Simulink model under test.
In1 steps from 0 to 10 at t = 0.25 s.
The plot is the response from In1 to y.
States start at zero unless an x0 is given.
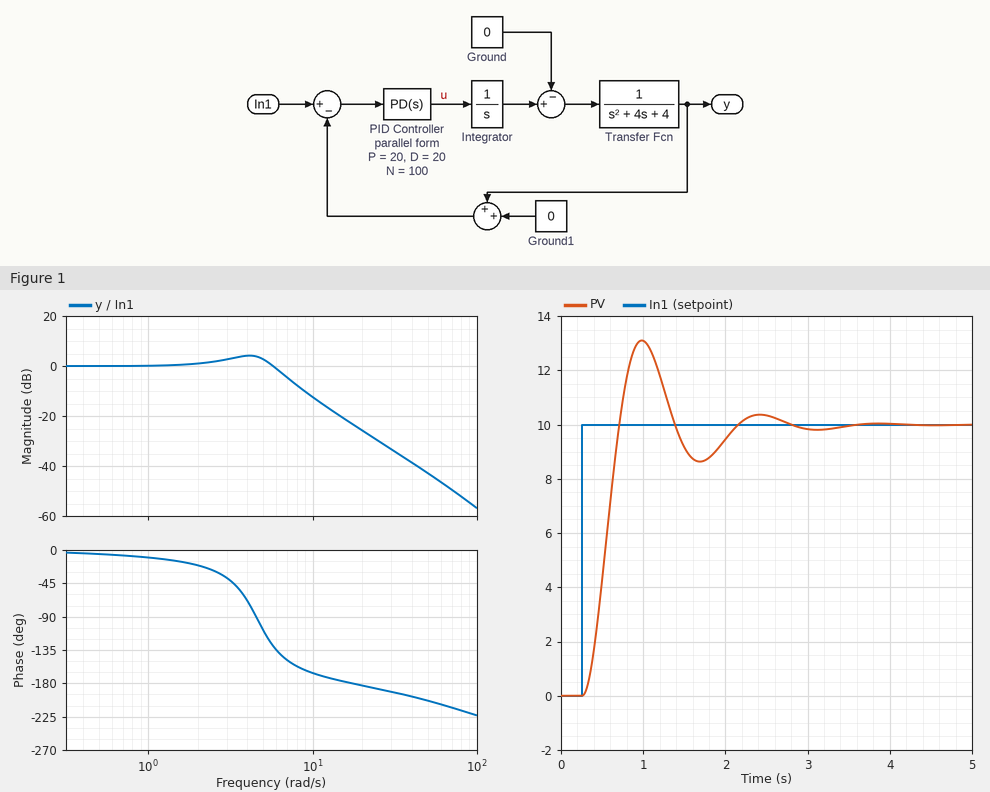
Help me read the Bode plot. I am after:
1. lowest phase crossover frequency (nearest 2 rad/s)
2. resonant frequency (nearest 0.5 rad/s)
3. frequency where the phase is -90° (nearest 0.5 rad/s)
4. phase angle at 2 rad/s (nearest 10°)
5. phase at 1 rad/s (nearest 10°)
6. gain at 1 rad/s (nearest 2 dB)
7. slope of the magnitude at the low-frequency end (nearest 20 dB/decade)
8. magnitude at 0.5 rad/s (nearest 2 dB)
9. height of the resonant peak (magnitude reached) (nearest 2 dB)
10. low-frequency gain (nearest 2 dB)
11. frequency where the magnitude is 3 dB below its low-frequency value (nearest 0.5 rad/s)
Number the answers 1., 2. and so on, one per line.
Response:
1. 18 rad/s
2. 4.0 rad/s
3. 4.5 rad/s
4. -20°
5. -10°
6. 0 dB
7. 0 dB/decade
8. 0 dB
9. 4 dB
10. 0 dB
11. 6.5 rad/s
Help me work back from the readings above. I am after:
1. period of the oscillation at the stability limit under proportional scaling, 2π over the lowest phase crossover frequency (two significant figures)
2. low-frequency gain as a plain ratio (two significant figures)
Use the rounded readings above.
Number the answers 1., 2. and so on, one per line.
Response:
1. 0.35 s
2. 1.0
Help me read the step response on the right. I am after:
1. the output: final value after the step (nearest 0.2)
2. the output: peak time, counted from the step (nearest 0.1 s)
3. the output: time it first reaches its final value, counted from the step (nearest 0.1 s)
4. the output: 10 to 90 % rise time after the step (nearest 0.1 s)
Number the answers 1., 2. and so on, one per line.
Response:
1. 10.0
2. 0.7 s
3. 0.5 s
4. 0.3 s
